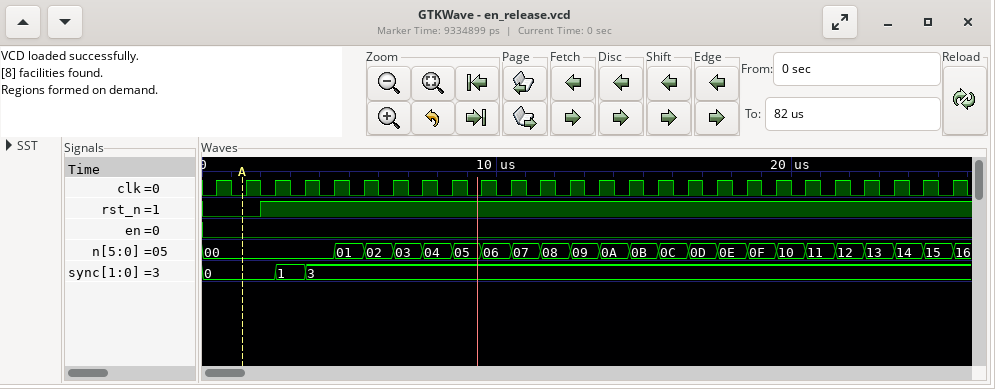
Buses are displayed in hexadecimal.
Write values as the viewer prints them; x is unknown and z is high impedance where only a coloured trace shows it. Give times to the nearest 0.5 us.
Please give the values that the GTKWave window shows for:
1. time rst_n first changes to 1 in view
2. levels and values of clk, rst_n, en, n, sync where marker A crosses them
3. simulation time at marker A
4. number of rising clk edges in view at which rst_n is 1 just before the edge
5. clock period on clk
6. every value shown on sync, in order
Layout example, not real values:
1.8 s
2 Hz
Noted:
2 us
clk=0, rst_n=0, en=0, n=00, sync=0
1.5 us
24
1 us
0, 1, 3
